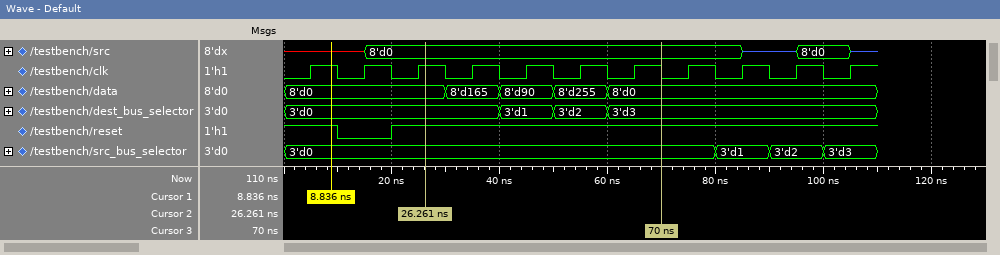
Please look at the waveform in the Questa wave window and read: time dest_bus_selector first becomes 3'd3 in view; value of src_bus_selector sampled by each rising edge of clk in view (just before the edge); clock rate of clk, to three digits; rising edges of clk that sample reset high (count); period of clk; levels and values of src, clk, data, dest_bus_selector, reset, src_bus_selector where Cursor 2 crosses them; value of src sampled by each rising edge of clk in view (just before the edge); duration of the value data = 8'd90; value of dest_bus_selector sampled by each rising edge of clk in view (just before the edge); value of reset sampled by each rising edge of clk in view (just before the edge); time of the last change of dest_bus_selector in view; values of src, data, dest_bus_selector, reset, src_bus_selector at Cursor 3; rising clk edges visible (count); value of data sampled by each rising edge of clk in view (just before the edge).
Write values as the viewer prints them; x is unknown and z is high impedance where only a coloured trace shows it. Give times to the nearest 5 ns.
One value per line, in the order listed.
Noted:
60 ns
3'd0, 3'd0, 3'd0, 3'd0, 3'd0, 3'd0, 3'd0, 3'd0, 3'd1, 3'd2, 3'd3
100 MHz
10
10 ns
src=8'd0, clk=1, data=8'd0, dest_bus_selector=3'd0, reset=1, src_bus_selector=3'd0
x, x, 8'd0, 8'd0, 8'd0, 8'd0, 8'd0, 8'd0, 8'd0, z, 8'd0
10 ns
3'd0, 3'd0, 3'd0, 3'd0, 3'd1, 3'd2, 3'd3, 3'd3, 3'd3, 3'd3, 3'd3
1 0 1 1 1 1 1 1 1 1 1
60 ns
src=8'd0, data=8'd0, dest_bus_selector=3'd3, reset=1, src_bus_selector=3'd0
11
8'd0, 8'd0, 8'd0, 8'd165, 8'd90, 8'd255, 8'd0, 8'd0, 8'd0, 8'd0, 8'd0
